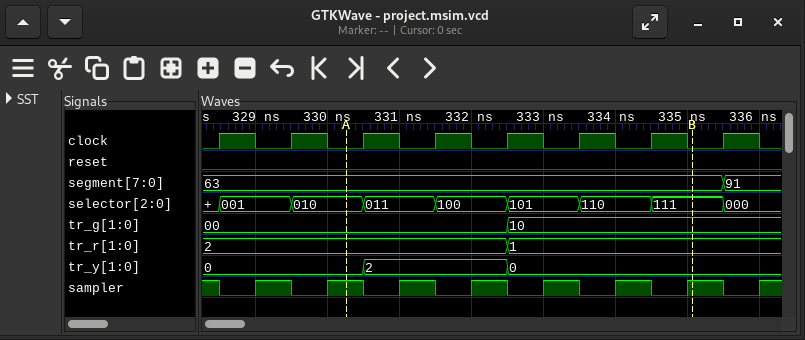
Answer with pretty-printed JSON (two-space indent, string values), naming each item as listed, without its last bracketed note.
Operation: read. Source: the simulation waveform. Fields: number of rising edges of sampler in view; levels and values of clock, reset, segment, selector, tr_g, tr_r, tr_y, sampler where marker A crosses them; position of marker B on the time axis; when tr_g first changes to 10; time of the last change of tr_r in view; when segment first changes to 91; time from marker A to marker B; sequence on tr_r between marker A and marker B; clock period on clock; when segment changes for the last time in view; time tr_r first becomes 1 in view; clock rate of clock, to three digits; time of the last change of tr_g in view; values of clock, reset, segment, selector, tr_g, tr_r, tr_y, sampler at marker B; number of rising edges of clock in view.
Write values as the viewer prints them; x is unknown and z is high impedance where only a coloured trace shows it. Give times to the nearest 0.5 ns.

{
  "number of rising edges of sampler in view": "8",
  "levels and values of clock, reset, segment, selector, tr_g, tr_r, tr_y, sampler where marker A crosses them": "clock=0, reset=0, segment=63, selector=010, tr_g=00, tr_r=2, tr_y=0, sampler=1",
  "position of marker B on the time axis": "335 ns",
  "when tr_g first changes to 10": "332.5 ns",
  "time of the last change of tr_r in view": "332.5 ns",
  "when segment first changes to 91": "335.5 ns",
  "time from marker A to marker B": "5 ns",
  "sequence on tr_r between marker A and marker B": "2, 1",
  "clock period on clock": "1 ns",
  "when segment changes for the last time in view": "335.5 ns",
  "time tr_r first becomes 1 in view": "332.5 ns",
  "clock rate of clock, to three digits": "1.00 GHz",
  "time of the last change of tr_g in view": "332.5 ns",
  "values of clock, reset, segment, selector, tr_g, tr_r, tr_y, sampler at marker B": "clock=0, reset=0, segment=63, selector=111, tr_g=10, tr_r=1, tr_y=0, sampler=1",
  "number of rising edges of clock in view": "8"
}
